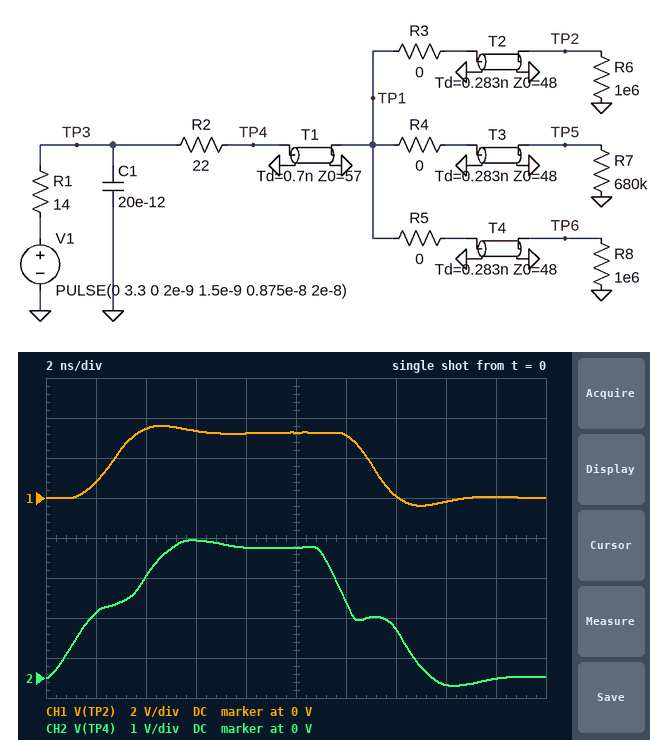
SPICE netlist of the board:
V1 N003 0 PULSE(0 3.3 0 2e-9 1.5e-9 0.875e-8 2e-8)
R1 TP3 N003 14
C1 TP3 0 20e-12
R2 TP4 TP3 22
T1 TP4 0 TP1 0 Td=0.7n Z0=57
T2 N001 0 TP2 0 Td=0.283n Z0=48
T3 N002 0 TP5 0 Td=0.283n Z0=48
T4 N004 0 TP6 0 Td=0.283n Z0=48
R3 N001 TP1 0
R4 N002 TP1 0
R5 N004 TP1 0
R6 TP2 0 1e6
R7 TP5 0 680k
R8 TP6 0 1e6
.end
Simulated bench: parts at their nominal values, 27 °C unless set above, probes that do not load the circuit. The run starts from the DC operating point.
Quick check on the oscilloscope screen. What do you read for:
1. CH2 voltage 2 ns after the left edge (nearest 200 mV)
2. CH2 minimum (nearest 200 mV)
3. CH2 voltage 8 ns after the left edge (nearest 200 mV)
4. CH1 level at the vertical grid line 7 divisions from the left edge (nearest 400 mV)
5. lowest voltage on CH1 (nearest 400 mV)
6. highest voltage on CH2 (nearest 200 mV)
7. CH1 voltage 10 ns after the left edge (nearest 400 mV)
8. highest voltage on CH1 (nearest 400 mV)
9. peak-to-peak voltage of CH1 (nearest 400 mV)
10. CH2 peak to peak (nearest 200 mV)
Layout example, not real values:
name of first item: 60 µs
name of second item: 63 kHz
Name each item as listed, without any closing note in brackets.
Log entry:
CH2 voltage 2 ns after the left edge: 1.6 V
CH2 minimum: -200 mV
CH2 voltage 8 ns after the left edge: 3.2 V
CH1 level at the vertical grid line 7 divisions from the left edge: 0 V
lowest voltage on CH1: -400 mV
highest voltage on CH2: 3.4 V
CH1 voltage 10 ns after the left edge: 3.2 V
highest voltage on CH1: 3.6 V
peak-to-peak voltage of CH1: 4.0 V
CH2 peak to peak: 3.6 V
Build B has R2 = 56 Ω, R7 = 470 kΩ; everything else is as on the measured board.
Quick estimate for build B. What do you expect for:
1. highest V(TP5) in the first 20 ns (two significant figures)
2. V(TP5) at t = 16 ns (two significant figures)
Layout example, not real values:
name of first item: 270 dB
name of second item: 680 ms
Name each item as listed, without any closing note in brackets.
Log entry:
highest V(TP5) in the first 20 ns: 3.2 V
V(TP5) at t = 16 ns: 330 mV
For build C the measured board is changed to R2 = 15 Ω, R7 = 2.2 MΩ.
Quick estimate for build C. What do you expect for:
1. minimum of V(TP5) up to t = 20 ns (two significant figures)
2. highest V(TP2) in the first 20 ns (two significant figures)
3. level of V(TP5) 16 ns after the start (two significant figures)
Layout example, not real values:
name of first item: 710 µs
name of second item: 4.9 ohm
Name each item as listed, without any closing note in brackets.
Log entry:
minimum of V(TP5) up to t = 20 ns: -710 mV
highest V(TP2) in the first 20 ns: 3.9 V
level of V(TP5) 16 ns after the start: -290 mV
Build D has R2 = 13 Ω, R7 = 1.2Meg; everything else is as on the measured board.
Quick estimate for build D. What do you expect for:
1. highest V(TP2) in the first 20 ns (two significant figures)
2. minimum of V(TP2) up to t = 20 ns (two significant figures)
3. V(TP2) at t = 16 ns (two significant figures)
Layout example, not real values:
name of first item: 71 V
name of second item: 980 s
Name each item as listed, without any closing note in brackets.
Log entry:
highest V(TP2) in the first 20 ns: 4.0 V
minimum of V(TP2) up to t = 20 ns: -810 mV
V(TP2) at t = 16 ns: -310 mV
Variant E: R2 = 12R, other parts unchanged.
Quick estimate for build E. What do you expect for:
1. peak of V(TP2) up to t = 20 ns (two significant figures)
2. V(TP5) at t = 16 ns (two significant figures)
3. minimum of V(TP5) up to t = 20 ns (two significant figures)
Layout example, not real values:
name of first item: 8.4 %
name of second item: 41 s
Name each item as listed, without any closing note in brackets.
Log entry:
peak of V(TP2) up to t = 20 ns: 4.1 V
V(TP5) at t = 16 ns: -320 mV
minimum of V(TP5) up to t = 20 ns: -860 mV
